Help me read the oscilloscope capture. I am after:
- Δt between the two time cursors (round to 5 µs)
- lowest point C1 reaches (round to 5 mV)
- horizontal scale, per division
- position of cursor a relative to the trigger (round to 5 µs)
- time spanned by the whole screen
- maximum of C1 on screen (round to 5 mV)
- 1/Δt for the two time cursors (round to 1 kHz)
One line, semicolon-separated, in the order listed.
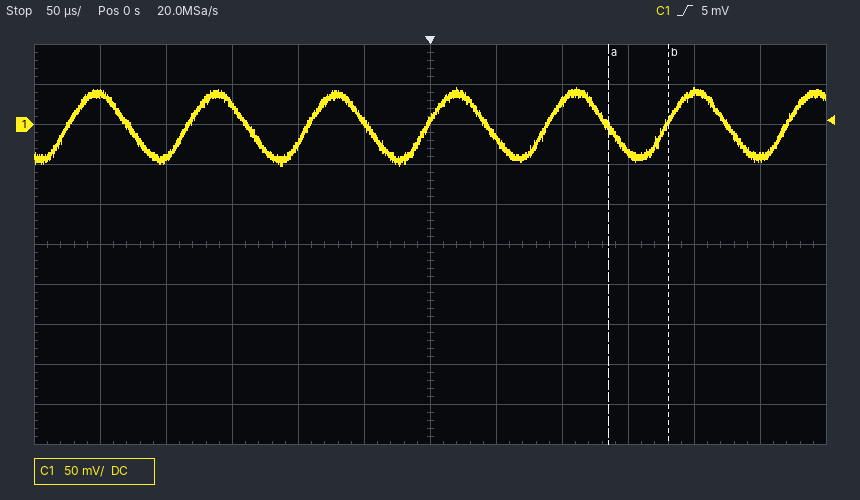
45 µs; -50 mV; 50 µs; +135 µs; 600 µs; 45 mV; 22 kHz
